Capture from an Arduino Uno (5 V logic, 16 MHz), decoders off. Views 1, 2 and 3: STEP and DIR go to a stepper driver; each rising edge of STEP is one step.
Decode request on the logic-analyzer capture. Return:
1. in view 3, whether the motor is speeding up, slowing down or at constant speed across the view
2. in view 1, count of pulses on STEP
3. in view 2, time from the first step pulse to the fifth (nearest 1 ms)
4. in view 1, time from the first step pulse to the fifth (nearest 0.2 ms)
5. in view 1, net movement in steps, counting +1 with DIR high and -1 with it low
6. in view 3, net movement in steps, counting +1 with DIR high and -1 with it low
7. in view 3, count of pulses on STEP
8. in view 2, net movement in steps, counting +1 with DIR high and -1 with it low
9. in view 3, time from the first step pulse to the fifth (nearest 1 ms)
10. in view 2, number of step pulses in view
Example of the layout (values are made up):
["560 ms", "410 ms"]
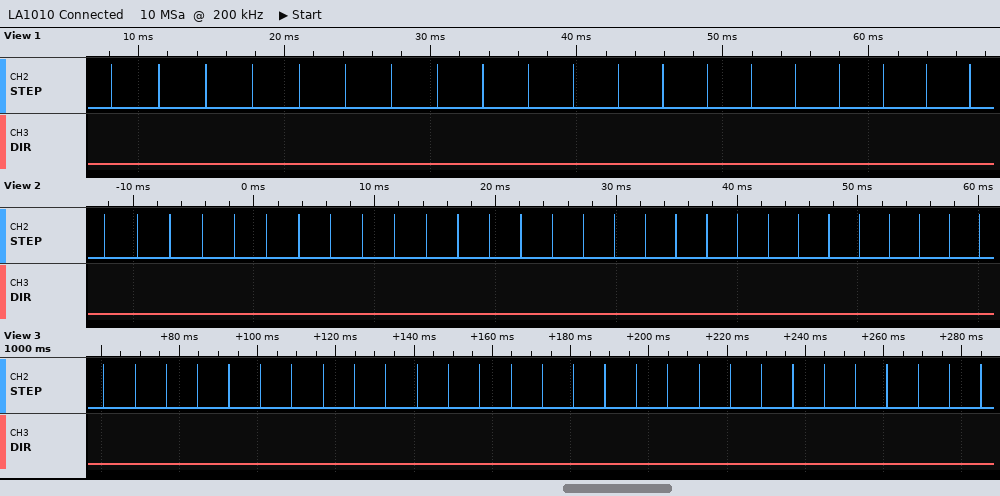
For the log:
["constant speed", "20", "11 ms", "12.8 ms", "-20", "-29", "29", "-29", "32 ms", "29"]
